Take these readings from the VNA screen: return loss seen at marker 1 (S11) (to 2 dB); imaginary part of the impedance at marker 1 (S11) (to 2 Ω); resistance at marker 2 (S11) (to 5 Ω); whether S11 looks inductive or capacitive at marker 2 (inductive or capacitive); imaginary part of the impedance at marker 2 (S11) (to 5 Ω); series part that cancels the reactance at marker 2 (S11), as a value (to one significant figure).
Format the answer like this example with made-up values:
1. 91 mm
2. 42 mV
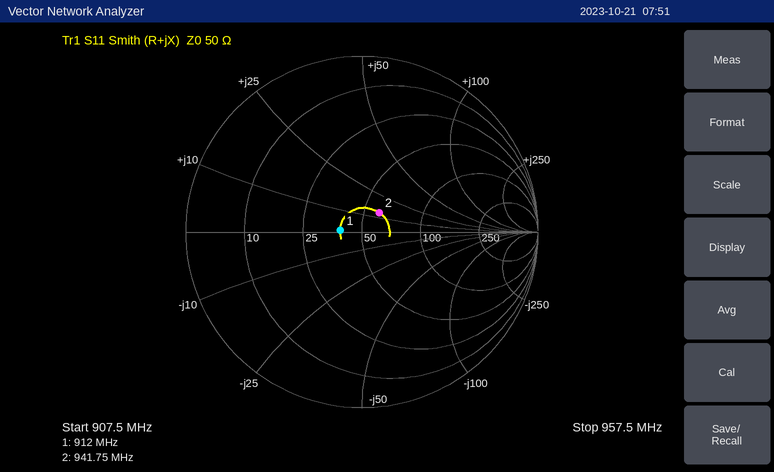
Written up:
1. 18 dB
2. 0 Ω
3. 60 Ω
4. inductive
5. +15 Ω
6. 10 pF
